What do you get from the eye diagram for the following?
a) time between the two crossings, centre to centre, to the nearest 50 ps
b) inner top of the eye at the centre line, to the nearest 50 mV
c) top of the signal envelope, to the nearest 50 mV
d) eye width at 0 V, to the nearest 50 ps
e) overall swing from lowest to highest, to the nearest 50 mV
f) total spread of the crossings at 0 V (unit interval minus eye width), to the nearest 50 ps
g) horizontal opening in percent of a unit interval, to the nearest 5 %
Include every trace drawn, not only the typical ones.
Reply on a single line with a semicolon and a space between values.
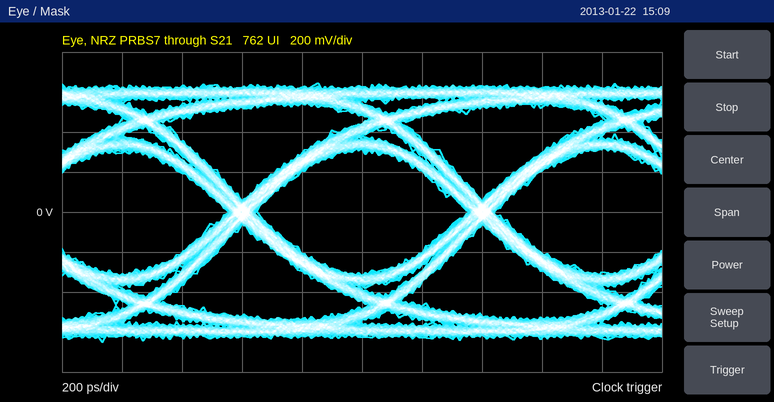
800 ps; 300 mV; 650 mV; 700 ps; 1.30 V; 100 ps; 90 %
